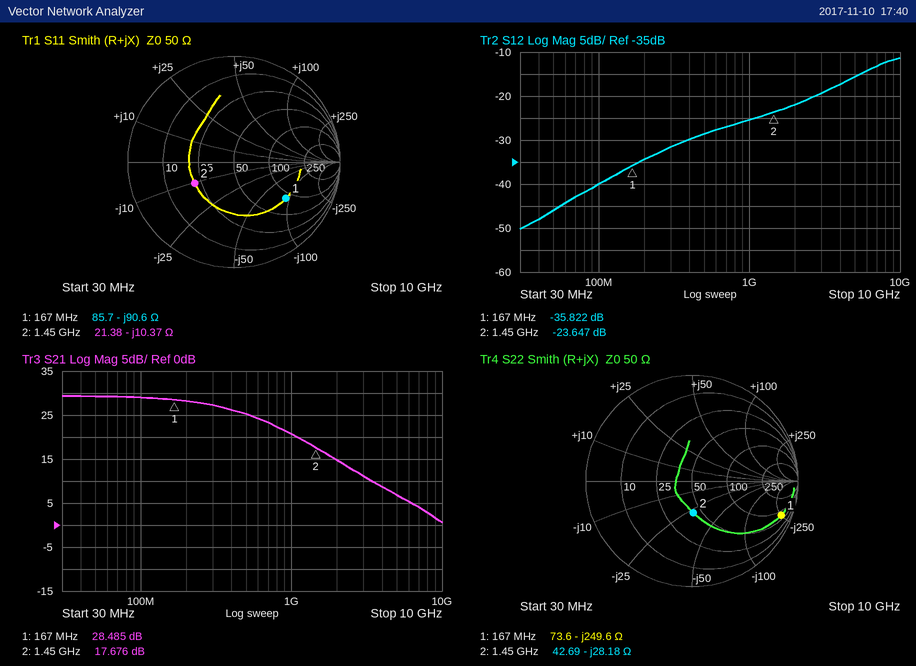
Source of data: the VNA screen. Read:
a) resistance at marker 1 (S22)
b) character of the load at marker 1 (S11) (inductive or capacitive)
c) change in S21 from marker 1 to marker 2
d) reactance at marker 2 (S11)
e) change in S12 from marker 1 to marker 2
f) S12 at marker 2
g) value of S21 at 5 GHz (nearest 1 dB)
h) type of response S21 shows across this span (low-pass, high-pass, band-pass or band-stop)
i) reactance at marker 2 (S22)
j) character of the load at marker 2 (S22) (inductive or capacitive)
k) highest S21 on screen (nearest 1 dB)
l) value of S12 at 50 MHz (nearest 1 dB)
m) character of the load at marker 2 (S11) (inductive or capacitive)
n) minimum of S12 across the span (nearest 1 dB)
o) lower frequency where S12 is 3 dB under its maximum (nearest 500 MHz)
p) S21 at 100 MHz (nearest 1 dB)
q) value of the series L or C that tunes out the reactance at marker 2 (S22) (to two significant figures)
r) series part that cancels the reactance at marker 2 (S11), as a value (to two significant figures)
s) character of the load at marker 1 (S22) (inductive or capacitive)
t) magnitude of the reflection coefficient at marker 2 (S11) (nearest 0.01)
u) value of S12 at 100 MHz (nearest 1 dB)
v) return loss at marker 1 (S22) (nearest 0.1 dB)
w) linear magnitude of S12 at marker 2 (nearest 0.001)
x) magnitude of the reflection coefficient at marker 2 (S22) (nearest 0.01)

73.6 Ω
capacitive
-10.809 dB
-10.37 Ω
12.175 dB
-23.647 dB
7 dB
low-pass
-28.18 Ω
capacitive
29 dB
-46 dB
capacitive
-50 dB
6.0 GHz
29 dB
3.1 nH
1.1 nH
capacitive
0.42
-40 dB
0.9 dB
0.066
0.30
